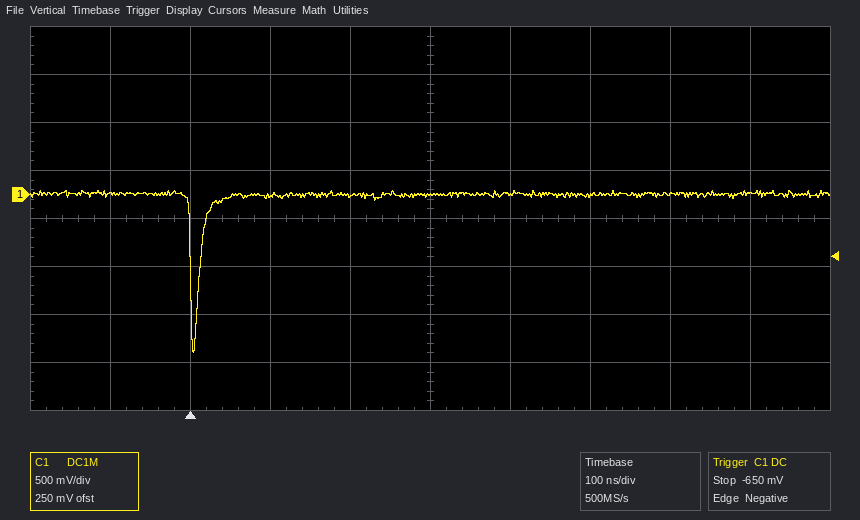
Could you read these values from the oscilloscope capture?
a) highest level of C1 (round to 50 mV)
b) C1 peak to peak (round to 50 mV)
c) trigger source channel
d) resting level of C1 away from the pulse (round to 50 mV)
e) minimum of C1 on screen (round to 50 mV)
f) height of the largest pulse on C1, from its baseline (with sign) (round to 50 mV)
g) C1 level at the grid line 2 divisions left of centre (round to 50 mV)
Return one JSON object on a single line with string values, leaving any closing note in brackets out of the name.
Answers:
{"highest level of C1": "50 mV", "C1 peak to peak": "1.70 V", "trigger source channel": "C1", "resting level of C1 away from the pulse": "0 mV", "minimum of C1 on screen": "-1.65 V", "height of the largest pulse on C1, from its baseline (with sign)": "-1.65 V", "C1 level at the grid line 2 divisions left of centre": "0 mV"}
